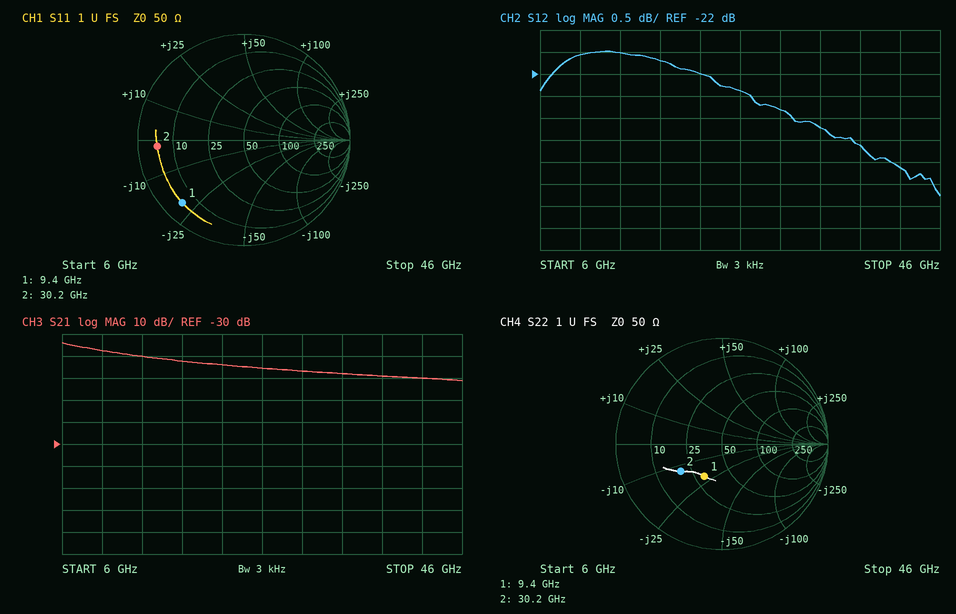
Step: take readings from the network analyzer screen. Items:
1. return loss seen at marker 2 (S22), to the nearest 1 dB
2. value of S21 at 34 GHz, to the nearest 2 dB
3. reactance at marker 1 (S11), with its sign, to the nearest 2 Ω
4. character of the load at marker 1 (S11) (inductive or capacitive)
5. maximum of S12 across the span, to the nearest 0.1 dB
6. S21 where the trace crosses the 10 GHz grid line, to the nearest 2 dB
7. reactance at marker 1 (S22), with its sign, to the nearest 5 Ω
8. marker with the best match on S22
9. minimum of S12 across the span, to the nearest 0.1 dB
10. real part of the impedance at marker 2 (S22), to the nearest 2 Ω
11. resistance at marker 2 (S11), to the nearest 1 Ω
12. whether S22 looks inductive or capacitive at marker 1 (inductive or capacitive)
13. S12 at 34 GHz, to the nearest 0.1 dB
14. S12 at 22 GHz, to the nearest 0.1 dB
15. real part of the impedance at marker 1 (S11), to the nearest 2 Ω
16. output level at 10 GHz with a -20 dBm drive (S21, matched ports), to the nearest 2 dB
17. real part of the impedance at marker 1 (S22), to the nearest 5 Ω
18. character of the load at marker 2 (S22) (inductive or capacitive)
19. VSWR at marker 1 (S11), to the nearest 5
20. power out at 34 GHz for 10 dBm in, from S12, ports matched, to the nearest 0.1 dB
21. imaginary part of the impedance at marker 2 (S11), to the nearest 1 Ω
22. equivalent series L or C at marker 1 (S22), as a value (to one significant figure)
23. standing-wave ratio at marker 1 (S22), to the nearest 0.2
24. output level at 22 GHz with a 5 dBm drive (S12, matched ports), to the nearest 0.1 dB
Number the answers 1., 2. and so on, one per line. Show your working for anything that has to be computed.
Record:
1. 7 dB
2. 2 dB
3. -20 Ω
4. capacitive
5. -21.5 dB
6. 12 dB
7. -20 Ω
8. marker 1
9. -24.8 dB
10. 20 Ω
11. 5 Ω
12. capacitive
13. -23.2 dB
14. -22.0 dB
15. 6 Ω
16. -20 dBm + (12 dB) = -8 dBm
17. 30 Ω
18. capacitive
19. 10
20. 10 dBm + (-23.2 dB) = -13.2 dBm
21. -2 Ω
22. C = 1/(2π × 9.4 GHz × 20 Ω) ≈ 847 fF, so 800 fF to one significant figure
23. 2.0
24. 5 dBm + (-22.0 dB) = -17.0 dBm
